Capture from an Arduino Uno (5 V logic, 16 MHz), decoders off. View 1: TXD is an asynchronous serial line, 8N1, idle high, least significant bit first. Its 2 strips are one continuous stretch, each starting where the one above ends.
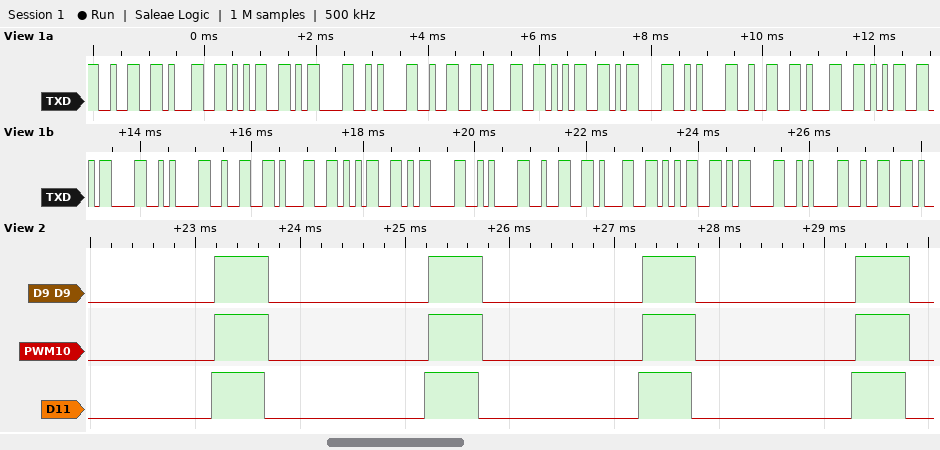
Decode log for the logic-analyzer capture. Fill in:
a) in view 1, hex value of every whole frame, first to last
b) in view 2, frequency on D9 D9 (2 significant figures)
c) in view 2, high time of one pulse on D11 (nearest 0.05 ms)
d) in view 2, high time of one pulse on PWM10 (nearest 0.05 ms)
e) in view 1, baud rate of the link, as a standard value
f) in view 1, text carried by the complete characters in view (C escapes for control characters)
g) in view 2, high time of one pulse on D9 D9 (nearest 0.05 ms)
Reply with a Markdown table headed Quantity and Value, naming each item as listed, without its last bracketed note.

| Quantity | Value |
|---|---|
| in view 1, hex value of every whole frame, first to last | 32 31 35 0D 0A 32 31 35 0D 0A 32 31 35 0D 0A 32 31 35 0D 0A 32 31 35 0D 0A 32 |
| in view 2, frequency on D9 D9 | 490 Hz |
| in view 2, high time of one pulse on D11 | 0.50 ms |
| in view 2, high time of one pulse on PWM10 | 0.50 ms |
| in view 1, baud rate of the link, as a standard value | 9600 baud |
| in view 1, text carried by the complete characters in view | "215\r\n215\r\n215\r\n215\r\n215\r\n2" |
| in view 2, high time of one pulse on D9 D9 | 0.50 ms |
